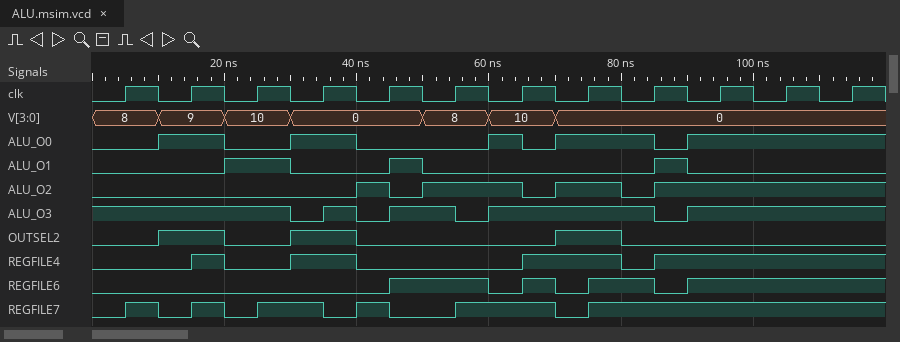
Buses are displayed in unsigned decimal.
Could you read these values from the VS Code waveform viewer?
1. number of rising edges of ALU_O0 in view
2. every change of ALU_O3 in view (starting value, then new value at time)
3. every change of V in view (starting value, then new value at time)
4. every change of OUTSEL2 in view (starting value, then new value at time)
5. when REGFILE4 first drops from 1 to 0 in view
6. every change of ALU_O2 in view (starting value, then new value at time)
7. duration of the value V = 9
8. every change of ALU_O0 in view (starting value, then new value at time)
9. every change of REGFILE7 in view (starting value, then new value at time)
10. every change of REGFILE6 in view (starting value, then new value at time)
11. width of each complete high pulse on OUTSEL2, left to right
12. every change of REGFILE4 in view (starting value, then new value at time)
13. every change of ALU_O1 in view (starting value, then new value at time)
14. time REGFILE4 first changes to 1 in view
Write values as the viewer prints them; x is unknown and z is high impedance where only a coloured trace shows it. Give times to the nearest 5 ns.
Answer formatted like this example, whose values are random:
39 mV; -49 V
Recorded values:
5; 1, 0 at 30 ns, 1 at 35 ns, 0 at 40 ns, 1 at 45 ns, 0 at 55 ns, 1 at 60 ns, 0 at 85 ns, 1 at 90 ns; 8, 9 at 10 ns, 10 at 20 ns, 0 at 30 ns, 8 at 50 ns, 10 at 60 ns, 0 at 70 ns; 0, 1 at 10 ns, 0 at 20 ns, 1 at 30 ns, 0 at 40 ns, 1 at 70 ns, 0 at 80 ns; 20 ns; 0, 1 at 40 ns, 0 at 45 ns, 1 at 50 ns, 0 at 65 ns, 1 at 70 ns, 0 at 80 ns, 1 at 85 ns; 10 ns; 0, 1 at 10 ns, 0 at 20 ns, 1 at 30 ns, 0 at 40 ns, 1 at 60 ns, 0 at 65 ns, 1 at 70 ns, 0 at 85 ns, 1 at 90 ns; 0, 1 at 5 ns, 0 at 10 ns, 1 at 15 ns, 0 at 20 ns, 1 at 25 ns, 0 at 35 ns, 1 at 40 ns, 0 at 45 ns, 1 at 55 ns, 0 at 70 ns, 1 at 75 ns; 0, 1 at 45 ns, 0 at 60 ns, 1 at 65 ns, 0 at 70 ns, 1 at 75 ns, 0 at 85 ns, 1 at 90 ns; 10 ns, 10 ns, 10 ns; 0, 1 at 15 ns, 0 at 20 ns, 1 at 30 ns, 0 at 40 ns, 1 at 65 ns, 0 at 80 ns, 1 at 85 ns; 0, 1 at 20 ns, 0 at 30 ns, 1 at 45 ns, 0 at 50 ns, 1 at 85 ns, 0 at 90 ns; 15 ns
